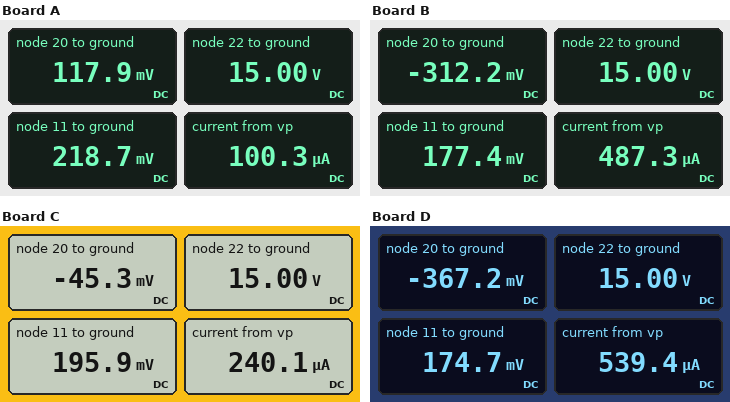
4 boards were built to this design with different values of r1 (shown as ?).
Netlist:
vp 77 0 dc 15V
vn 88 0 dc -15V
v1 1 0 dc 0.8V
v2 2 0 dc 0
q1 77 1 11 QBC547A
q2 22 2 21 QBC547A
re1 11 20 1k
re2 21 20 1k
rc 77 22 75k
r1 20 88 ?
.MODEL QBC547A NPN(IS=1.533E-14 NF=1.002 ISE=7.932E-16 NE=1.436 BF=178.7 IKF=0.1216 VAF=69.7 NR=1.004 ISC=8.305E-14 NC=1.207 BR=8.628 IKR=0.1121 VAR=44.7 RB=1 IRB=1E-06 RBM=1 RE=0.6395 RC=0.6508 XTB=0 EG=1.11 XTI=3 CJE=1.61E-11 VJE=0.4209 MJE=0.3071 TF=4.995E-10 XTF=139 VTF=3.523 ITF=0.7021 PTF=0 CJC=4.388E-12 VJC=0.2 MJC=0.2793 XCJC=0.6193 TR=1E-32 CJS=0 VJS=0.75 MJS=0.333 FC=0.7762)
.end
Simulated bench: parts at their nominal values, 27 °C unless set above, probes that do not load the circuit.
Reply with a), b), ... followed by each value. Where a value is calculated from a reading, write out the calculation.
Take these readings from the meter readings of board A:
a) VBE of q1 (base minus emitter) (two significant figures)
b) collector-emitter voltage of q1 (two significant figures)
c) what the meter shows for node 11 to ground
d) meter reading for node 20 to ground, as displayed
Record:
a) 800 mV - 218.7 mV = 580 mV
b) 15 V - 218.7 mV = 15 V
c) 218.7 mV
d) 117.9 mV
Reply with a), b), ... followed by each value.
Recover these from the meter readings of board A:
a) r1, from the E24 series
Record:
a) 150 kΩ
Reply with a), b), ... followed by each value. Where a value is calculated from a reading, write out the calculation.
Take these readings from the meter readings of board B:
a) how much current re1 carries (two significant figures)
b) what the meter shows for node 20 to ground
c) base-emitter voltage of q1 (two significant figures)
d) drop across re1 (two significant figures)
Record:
a) (177.4 mV - (-312.2 mV)) / 1 kΩ = 490 µA
b) -312.2 mV
c) 800 mV - 177.4 mV = 620 mV
d) 177.4 mV - (-312.2 mV) = 490 mV
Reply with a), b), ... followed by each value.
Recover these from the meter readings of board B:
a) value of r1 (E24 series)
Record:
a) 30 kΩ
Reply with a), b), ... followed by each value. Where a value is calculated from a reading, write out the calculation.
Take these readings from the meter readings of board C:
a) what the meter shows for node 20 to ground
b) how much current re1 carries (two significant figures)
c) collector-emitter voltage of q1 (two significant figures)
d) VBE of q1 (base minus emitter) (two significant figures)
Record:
a) -45.3 mV
b) (195.9 mV - (-45.3 mV)) / 1 kΩ = 240 µA
c) 15 V - 195.9 mV = 15 V
d) 800 mV - 195.9 mV = 600 mV
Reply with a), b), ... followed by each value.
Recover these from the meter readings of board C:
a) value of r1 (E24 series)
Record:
a) 62 kΩ
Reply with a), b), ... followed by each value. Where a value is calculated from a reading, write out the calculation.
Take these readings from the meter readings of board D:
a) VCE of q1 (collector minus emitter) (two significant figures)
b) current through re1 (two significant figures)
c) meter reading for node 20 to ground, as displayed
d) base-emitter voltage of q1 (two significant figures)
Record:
a) 15 V - 174.7 mV = 15 V
b) (174.7 mV - (-367.2 mV)) / 1 kΩ = 540 µA
c) -367.2 mV
d) 800 mV - 174.7 mV = 630 mV
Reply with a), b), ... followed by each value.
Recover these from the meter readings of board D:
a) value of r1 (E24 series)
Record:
a) 27 kΩ
